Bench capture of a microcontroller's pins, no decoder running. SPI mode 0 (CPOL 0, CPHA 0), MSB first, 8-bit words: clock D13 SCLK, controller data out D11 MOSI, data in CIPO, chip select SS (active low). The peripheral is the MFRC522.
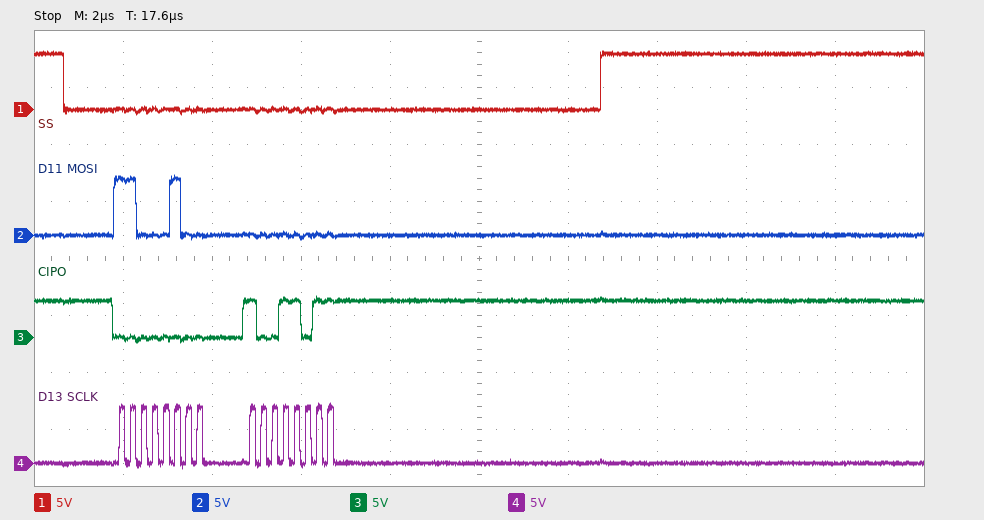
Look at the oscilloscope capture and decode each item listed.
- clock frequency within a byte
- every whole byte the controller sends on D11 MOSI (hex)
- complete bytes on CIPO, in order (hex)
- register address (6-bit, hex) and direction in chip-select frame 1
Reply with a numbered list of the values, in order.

1. 4 MHz
2. 0xC4 0x00
3. 0x00 0x9B
4. 0x22 read
